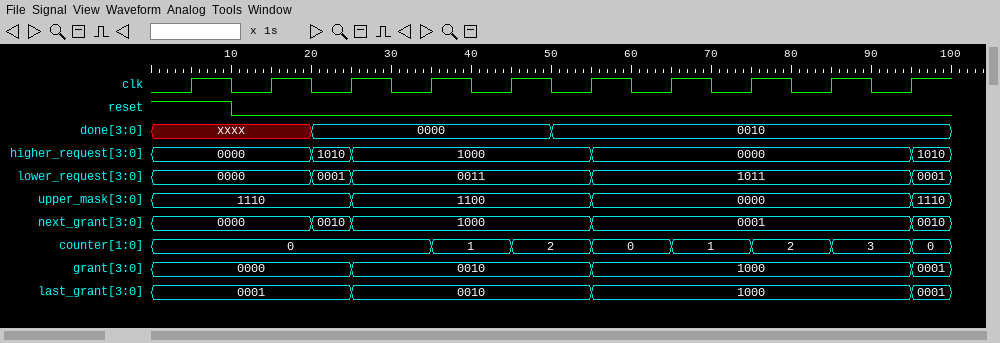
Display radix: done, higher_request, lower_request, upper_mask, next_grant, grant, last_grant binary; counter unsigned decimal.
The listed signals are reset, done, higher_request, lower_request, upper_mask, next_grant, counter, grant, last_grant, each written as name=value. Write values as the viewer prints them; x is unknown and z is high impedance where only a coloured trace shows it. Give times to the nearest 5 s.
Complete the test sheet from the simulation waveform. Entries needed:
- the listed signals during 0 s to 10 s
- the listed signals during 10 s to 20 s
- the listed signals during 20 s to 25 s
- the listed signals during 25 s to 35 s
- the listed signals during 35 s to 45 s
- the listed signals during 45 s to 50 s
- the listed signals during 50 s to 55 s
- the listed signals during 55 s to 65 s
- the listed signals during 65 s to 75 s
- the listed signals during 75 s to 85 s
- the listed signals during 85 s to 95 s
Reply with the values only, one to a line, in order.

reset=1, done=xxxx, higher_request=0000, lower_request=0000, upper_mask=1110, next_grant=0000, counter=0, grant=0000, last_grant=0001
reset=0, done=xxxx, higher_request=0000, lower_request=0000, upper_mask=1110, next_grant=0000, counter=0, grant=0000, last_grant=0001
reset=0, done=0000, higher_request=1010, lower_request=0001, upper_mask=1110, next_grant=0010, counter=0, grant=0000, last_grant=0001
reset=0, done=0000, higher_request=1000, lower_request=0011, upper_mask=1100, next_grant=1000, counter=0, grant=0010, last_grant=0010
reset=0, done=0000, higher_request=1000, lower_request=0011, upper_mask=1100, next_grant=1000, counter=1, grant=0010, last_grant=0010
reset=0, done=0000, higher_request=1000, lower_request=0011, upper_mask=1100, next_grant=1000, counter=2, grant=0010, last_grant=0010
reset=0, done=0010, higher_request=1000, lower_request=0011, upper_mask=1100, next_grant=1000, counter=2, grant=0010, last_grant=0010
reset=0, done=0010, higher_request=0000, lower_request=1011, upper_mask=0000, next_grant=0001, counter=0, grant=1000, last_grant=1000
reset=0, done=0010, higher_request=0000, lower_request=1011, upper_mask=0000, next_grant=0001, counter=1, grant=1000, last_grant=1000
reset=0, done=0010, higher_request=0000, lower_request=1011, upper_mask=0000, next_grant=0001, counter=2, grant=1000, last_grant=1000
reset=0, done=0010, higher_request=0000, lower_request=1011, upper_mask=0000, next_grant=0001, counter=3, grant=1000, last_grant=1000
